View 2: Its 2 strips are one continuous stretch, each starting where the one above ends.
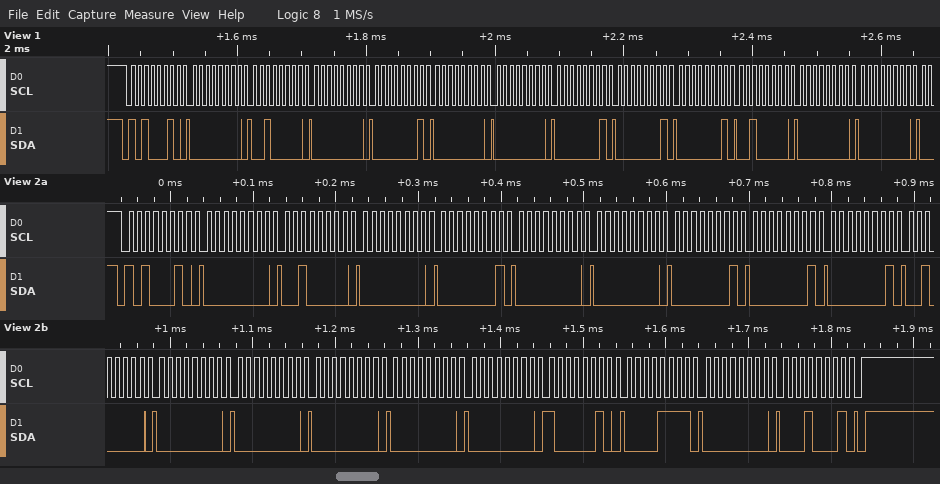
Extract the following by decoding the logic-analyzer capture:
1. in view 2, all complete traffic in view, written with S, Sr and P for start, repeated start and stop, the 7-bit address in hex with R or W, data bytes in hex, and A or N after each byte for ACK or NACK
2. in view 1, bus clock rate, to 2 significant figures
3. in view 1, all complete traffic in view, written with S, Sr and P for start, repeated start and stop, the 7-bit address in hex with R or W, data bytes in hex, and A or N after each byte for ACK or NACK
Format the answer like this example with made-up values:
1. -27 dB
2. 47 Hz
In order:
1. S 51W A 00 A 20 A 00 A 01 A 00 A 00 A 01 A 01 A 01 A 20 A 00 A 00 A 00 A 00 A 00 A 82 A 0F A 00 A 11 A P
2. 100 kHz
3. S 51W A 00 A 20 A 00 A 01 A 00 A 00 A 01 A 01 A 01 A 20 A 00 A 00 A
